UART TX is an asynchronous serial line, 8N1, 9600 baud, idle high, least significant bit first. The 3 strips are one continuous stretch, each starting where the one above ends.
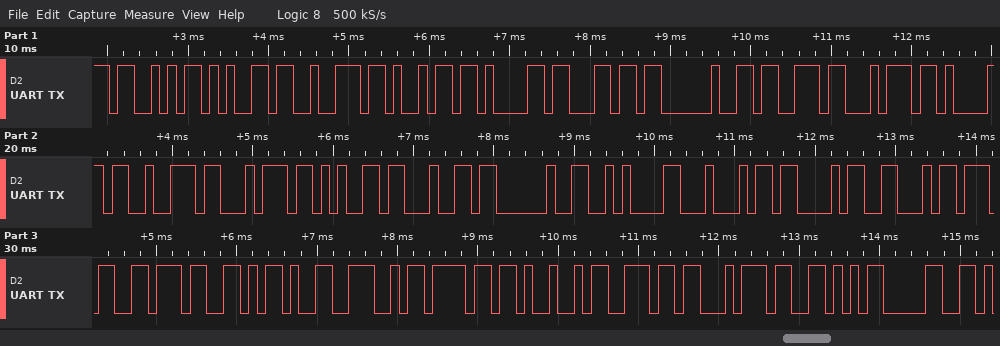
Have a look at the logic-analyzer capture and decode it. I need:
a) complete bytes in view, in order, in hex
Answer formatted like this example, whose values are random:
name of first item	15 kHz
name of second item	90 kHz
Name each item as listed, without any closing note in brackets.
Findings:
complete bytes in view, in order, in hex	53 65 72 69 61 6C 20 73 74 61 72 74 65 64 20 0A 44 43 46 37 37 2D 4E 6F 49 6E 74 56 30
